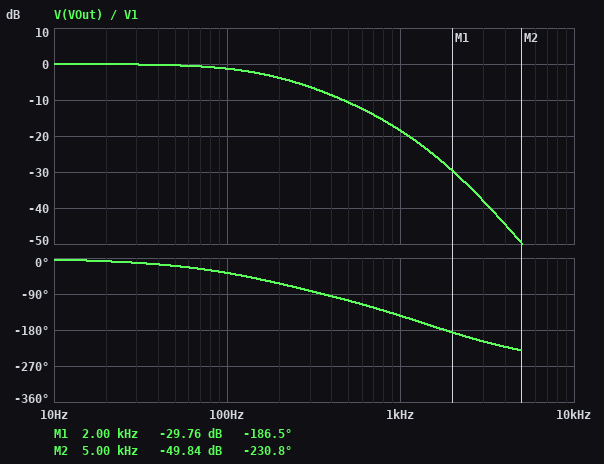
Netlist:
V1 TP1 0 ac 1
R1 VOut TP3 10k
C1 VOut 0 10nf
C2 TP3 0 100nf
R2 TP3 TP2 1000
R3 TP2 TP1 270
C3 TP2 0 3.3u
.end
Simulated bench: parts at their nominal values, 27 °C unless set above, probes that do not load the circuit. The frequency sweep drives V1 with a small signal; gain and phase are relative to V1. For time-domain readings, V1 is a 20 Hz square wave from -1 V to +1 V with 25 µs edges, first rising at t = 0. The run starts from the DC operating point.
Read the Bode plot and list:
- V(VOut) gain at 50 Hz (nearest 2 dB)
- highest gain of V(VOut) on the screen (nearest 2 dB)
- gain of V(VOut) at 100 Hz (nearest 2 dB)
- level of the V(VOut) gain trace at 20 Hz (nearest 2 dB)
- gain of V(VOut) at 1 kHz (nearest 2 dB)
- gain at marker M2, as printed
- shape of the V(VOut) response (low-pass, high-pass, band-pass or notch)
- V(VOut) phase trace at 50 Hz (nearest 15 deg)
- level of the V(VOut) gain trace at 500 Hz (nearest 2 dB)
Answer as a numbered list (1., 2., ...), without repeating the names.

1. 0 dB
2. 0 dB
3. -2 dB
4. 0 dB
5. -18 dB
6. -49.84 dB
7. low-pass
8. -15 deg
9. -10 dB
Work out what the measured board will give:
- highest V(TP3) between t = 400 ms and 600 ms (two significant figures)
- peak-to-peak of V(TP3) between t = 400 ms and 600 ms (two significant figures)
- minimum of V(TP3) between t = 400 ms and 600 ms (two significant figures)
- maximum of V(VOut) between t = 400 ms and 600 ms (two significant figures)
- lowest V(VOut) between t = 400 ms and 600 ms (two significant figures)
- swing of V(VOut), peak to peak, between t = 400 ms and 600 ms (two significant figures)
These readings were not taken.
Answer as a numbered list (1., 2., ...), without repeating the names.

1. 1.0 V
2. 2.0 V
3. -1.0 V
4. 1.0 V
5. -1.0 V
6. 2.0 V
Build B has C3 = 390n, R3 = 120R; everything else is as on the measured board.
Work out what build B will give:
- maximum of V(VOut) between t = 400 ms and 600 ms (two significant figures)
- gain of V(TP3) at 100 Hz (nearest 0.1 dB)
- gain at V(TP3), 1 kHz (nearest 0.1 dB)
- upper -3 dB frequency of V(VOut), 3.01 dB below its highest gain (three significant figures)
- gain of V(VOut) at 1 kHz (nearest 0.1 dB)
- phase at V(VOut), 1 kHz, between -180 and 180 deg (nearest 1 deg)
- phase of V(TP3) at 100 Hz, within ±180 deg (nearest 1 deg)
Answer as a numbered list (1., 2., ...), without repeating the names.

1. 1.0 V
2. 0 dB
3. -2.6 dB
4. 836 Hz
5. -4.0 dB
6. -84 deg
7. -6 deg
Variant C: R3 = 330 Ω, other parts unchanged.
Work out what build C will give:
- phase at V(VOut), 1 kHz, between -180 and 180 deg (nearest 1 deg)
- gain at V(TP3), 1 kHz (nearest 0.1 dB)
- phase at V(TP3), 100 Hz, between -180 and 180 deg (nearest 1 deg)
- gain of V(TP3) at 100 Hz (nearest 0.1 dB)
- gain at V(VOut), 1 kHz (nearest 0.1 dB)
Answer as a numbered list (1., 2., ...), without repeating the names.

1. -146 deg
2. -18.8 dB
3. -39 deg
4. -1.8 dB
5. -20.2 dB
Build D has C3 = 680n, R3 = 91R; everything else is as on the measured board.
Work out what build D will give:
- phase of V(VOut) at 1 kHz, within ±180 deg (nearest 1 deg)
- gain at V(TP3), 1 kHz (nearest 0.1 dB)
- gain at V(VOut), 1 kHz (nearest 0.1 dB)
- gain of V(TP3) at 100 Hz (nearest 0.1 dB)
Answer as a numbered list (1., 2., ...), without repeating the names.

1. -88 deg
2. -2.7 dB
3. -4.2 dB
4. 0 dB
